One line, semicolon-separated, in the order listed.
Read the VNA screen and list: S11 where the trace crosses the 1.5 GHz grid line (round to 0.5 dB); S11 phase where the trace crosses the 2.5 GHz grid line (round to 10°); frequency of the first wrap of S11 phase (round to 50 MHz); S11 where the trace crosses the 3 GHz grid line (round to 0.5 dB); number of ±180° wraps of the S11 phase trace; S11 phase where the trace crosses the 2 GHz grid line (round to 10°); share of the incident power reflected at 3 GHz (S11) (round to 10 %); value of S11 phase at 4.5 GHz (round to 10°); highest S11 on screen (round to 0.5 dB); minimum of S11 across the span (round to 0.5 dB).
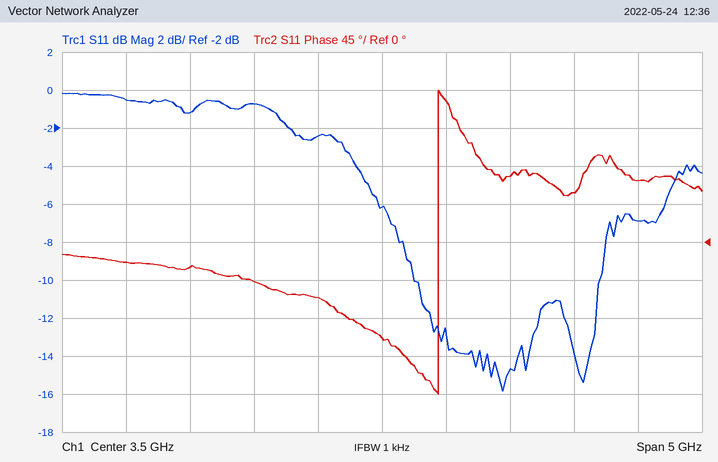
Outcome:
-0.5 dB; -50°; 3.95 GHz; -2.5 dB; 1; -30°; 60 %; 80°; 0.0 dB; -16.0 dB
